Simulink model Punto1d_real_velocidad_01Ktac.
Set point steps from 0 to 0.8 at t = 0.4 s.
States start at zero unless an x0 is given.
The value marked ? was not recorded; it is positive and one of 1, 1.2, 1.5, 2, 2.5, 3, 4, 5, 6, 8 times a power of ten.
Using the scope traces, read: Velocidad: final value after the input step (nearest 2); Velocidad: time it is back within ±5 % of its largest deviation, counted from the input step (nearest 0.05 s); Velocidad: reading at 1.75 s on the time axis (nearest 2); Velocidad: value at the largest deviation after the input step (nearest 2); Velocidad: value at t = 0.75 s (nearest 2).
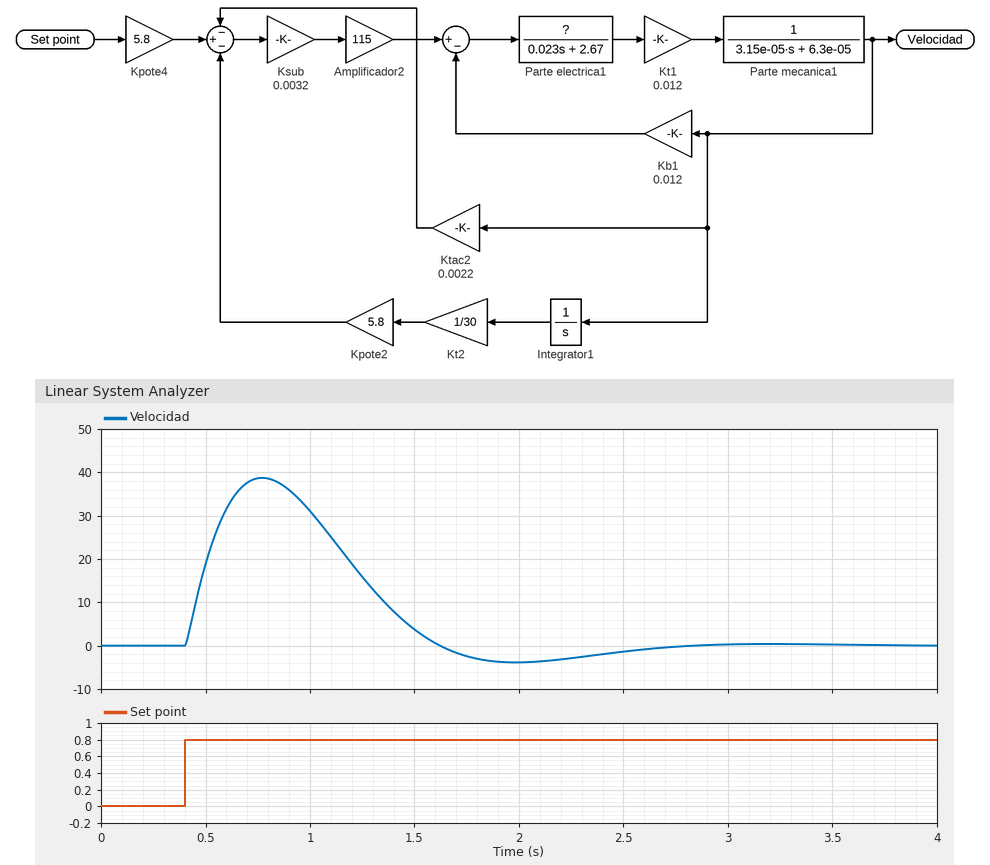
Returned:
0
2.00 s
-2
38
38
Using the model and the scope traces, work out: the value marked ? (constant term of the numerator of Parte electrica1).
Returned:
1
